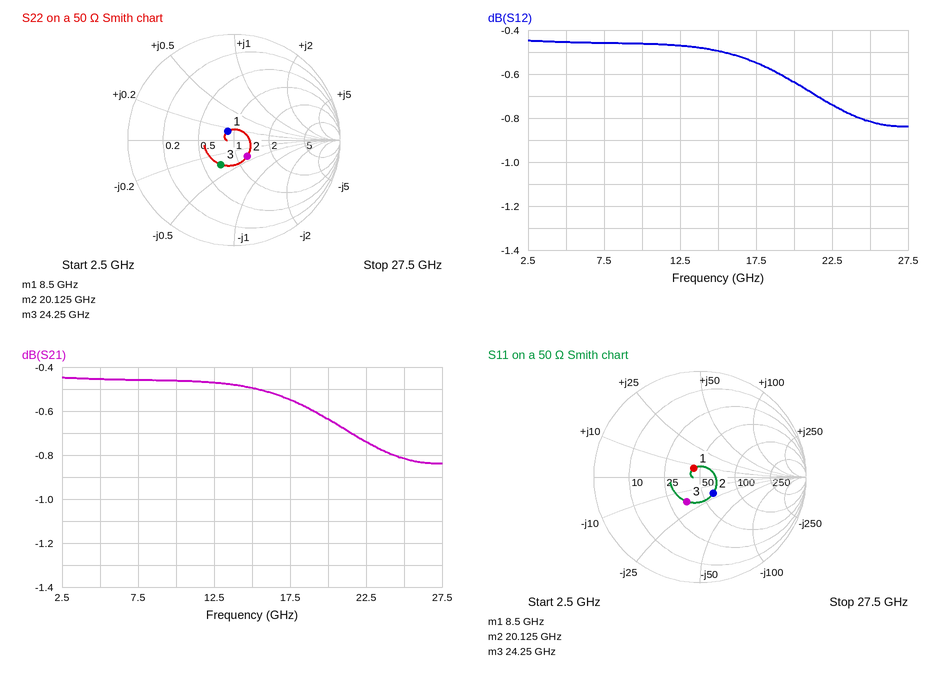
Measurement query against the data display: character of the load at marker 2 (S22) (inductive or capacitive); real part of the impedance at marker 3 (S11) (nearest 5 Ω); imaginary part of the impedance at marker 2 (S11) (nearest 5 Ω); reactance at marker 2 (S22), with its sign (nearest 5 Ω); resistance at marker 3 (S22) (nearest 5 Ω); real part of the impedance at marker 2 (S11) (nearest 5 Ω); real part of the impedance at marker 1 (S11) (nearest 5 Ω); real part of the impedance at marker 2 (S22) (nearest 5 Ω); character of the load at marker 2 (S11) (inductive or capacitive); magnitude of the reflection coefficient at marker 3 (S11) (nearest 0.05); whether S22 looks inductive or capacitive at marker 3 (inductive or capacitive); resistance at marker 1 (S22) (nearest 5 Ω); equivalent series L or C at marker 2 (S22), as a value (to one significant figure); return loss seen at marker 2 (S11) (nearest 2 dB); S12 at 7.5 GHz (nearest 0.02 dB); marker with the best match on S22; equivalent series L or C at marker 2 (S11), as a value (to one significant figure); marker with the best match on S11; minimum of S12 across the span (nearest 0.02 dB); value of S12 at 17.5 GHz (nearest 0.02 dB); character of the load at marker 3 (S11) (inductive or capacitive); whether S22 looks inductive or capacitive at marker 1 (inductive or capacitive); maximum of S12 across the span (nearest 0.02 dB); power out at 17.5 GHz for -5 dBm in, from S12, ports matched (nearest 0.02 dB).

capacitive
35 Ω
-20 Ω
-20 Ω
35 Ω
60 Ω
45 Ω
60 Ω
capacitive
0.25
capacitive
45 Ω
400 fF
14 dB
-0.46 dB
marker 1
400 fF
marker 1
-0.84 dB
-0.54 dB
capacitive
inductive
-0.44 dB
-5.54 dBm
